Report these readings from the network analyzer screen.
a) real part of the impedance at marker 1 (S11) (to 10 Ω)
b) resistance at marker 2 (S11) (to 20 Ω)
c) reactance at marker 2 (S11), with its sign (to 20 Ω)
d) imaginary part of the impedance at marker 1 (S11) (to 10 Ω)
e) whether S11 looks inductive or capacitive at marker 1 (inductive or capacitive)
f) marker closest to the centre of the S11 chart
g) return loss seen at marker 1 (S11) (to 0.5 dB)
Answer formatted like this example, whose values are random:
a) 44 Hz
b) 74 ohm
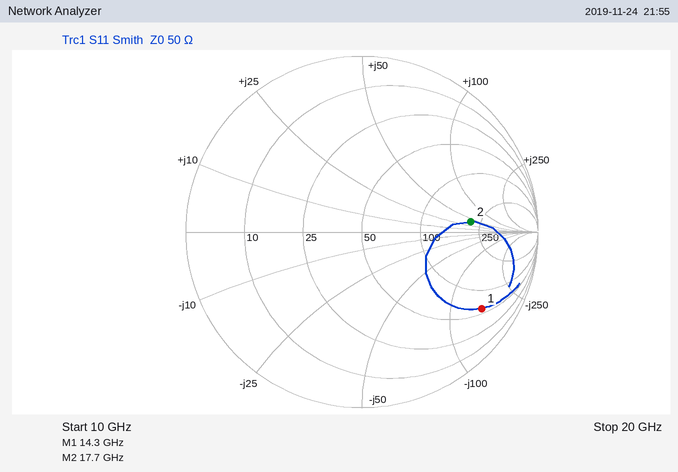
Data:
a) 60 Ω
b) 200 Ω
c) +40 Ω
d) -150 Ω
e) capacitive
f) marker 2
g) 2.0 dB
